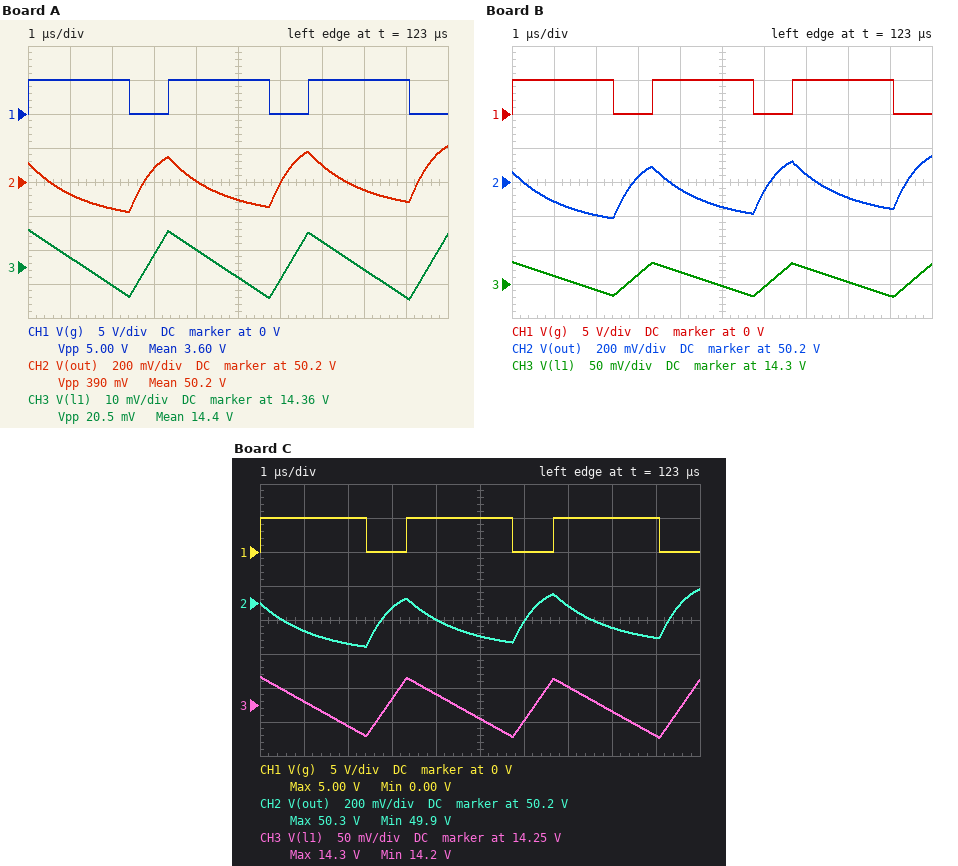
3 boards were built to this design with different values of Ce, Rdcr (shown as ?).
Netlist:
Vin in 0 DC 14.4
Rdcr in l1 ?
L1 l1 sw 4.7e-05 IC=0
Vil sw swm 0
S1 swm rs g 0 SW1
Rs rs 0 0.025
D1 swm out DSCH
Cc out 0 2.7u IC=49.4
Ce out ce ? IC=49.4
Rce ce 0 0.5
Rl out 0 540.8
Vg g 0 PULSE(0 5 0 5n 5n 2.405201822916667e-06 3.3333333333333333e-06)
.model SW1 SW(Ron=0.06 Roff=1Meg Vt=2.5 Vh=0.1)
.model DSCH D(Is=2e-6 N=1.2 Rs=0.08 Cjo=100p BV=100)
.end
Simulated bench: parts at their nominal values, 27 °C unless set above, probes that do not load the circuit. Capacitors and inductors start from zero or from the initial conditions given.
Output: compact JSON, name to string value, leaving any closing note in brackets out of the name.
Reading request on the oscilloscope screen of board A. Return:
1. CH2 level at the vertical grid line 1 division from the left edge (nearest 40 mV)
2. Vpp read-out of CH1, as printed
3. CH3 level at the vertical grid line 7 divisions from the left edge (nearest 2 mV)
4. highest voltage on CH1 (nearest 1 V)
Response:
{"CH2 level at the vertical grid line 1 division from the left edge": "50.12 V", "Vpp read-out of CH1, as printed": "5.00 V", "CH3 level at the vertical grid line 7 divisions from the left edge": "14.368 V", "highest voltage on CH1": "5 V"}
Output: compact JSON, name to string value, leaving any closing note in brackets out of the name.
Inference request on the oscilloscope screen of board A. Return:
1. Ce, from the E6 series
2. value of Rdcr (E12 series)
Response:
{"Ce, from the E6 series": "33 µF", "value of Rdcr": "0.027 Ω"}
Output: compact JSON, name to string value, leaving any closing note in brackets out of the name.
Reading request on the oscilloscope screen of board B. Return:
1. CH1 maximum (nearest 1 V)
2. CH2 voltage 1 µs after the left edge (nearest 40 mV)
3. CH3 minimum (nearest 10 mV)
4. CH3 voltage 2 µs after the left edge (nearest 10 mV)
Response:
{"CH1 maximum": "5 V", "CH2 voltage 1 µs after the left edge": "50.08 V", "CH3 minimum": "14.28 V", "CH3 voltage 2 µs after the left edge": "14.29 V"}
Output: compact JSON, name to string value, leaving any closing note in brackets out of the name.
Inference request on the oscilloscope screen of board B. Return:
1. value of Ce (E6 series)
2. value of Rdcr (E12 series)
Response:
{"value of Ce": "33 µF", "value of Rdcr": "0.068 Ω"}
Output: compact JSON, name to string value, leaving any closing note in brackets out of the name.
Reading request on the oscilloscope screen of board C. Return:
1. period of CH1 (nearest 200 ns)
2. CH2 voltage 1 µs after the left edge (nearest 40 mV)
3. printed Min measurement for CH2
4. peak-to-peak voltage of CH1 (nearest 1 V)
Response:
{"period of CH1": "3.4 µs", "CH2 voltage 1 µs after the left edge": "50.04 V", "printed Min measurement for CH2": "49.9 V", "peak-to-peak voltage of CH1": "5 V"}
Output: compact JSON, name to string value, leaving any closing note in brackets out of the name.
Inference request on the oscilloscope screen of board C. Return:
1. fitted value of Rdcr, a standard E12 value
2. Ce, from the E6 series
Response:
{"fitted value of Rdcr, a standard E12 value": "0.12 Ω", "Ce, from the E6 series": "33 µF"}
